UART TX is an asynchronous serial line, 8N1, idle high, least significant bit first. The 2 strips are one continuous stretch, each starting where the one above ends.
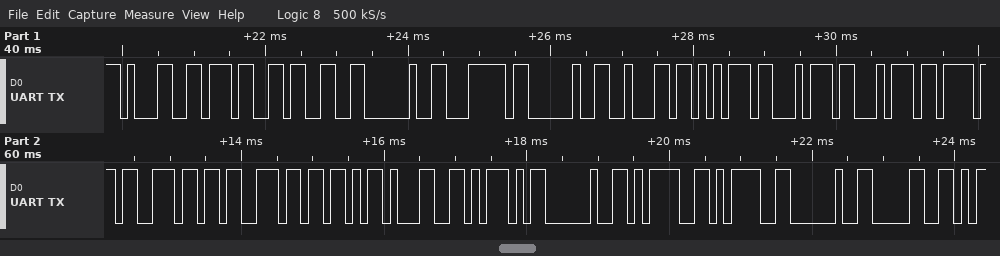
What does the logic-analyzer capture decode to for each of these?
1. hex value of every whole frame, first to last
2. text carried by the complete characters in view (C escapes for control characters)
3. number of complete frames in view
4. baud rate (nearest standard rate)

31 37 33 20 7C 20 62 75 74 74 6F 6E 73 5B 31 5D 20 3D 3D 20 30
"173 | buttons[1] == 0"
21
9600 baud
